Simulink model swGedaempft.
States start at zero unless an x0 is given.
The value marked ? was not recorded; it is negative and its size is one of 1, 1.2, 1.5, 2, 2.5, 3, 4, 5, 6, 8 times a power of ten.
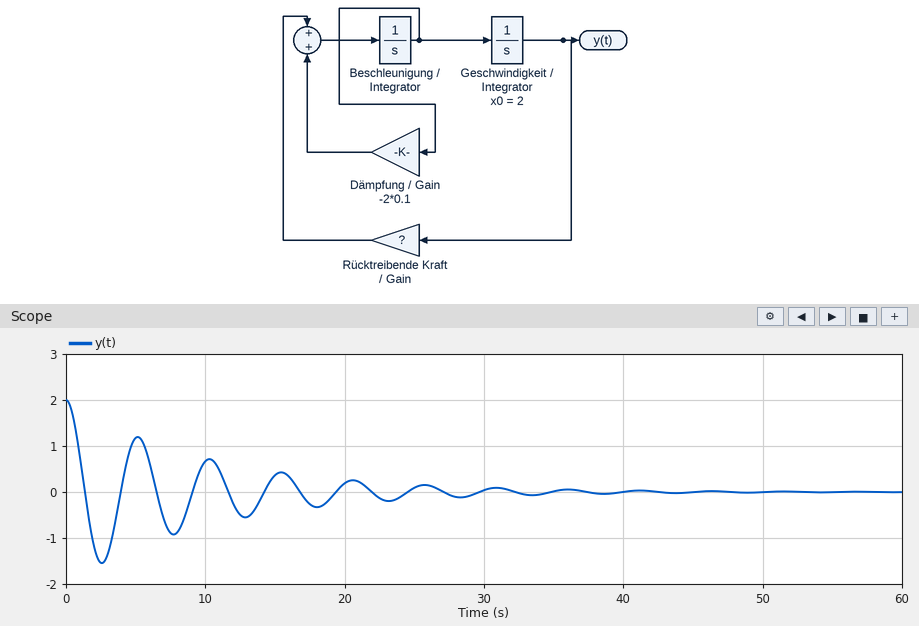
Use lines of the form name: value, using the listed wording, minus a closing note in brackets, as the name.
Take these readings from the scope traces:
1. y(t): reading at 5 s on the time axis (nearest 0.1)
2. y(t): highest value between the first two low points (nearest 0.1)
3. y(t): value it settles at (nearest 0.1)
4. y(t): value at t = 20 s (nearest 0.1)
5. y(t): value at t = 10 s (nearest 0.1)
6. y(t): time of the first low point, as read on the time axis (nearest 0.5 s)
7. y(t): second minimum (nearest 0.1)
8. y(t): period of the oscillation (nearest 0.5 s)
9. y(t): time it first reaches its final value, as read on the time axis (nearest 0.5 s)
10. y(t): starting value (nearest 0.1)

y(t): reading at 5 s on the time axis: 1.2
y(t): highest value between the first two low points: 1.2
y(t): value it settles at: 0.0
y(t): value at t = 20 s: 0.2
y(t): value at t = 10 s: 0.7
y(t): time of the first low point, as read on the time axis: 2.5 s
y(t): second minimum: -0.9
y(t): period of the oscillation: 5.0 s
y(t): time it first reaches its final value, as read on the time axis: 1.5 s
y(t): starting value: 2.0
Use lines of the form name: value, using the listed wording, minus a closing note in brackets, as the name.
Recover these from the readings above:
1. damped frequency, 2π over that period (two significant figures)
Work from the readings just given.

damped frequency, 2π over that period: 1.3 rad/s
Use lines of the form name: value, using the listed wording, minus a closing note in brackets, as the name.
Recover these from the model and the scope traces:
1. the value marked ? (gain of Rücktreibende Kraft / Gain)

the value marked ?: -1.5
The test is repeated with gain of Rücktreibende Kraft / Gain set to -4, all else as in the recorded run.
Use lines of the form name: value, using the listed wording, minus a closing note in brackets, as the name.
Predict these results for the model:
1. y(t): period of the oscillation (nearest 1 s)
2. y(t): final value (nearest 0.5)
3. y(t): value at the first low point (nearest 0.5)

y(t): period of the oscillation: 3 s
y(t): final value: 0.0
y(t): value at the first low point: -1.5
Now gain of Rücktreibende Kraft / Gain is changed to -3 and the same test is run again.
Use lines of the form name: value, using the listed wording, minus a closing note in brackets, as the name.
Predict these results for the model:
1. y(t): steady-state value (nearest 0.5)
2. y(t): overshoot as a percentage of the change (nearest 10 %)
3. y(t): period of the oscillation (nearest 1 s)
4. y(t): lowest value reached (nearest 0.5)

y(t): steady-state value: 0.0
y(t): overshoot as a percentage of the change: 80 %
y(t): period of the oscillation: 4 s
y(t): lowest value reached: -1.5
